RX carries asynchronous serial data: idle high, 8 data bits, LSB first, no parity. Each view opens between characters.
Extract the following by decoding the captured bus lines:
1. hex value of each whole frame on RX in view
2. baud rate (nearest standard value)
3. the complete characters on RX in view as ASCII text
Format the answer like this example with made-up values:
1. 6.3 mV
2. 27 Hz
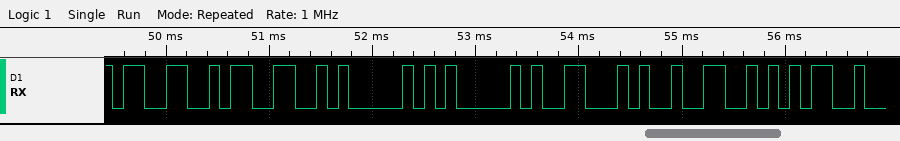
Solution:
1. 33, 33, 41, 41, 46, 32, 35
2. 9600 baud
3. "33AAF25"
